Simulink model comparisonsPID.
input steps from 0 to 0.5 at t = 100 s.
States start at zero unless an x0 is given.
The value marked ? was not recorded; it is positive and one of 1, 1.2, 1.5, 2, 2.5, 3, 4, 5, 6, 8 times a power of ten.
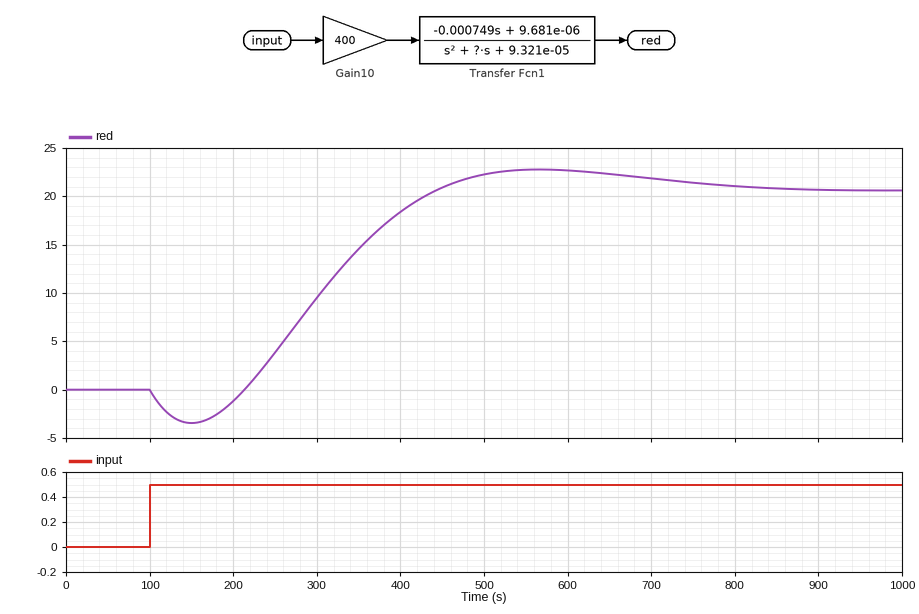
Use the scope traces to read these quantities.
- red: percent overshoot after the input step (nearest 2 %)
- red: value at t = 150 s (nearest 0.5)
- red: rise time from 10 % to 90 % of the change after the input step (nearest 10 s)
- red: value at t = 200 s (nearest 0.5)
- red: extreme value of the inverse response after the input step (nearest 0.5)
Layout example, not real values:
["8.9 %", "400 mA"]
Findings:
["10 %", "-3.5", "170 s", "-1.0", "-3.5"]
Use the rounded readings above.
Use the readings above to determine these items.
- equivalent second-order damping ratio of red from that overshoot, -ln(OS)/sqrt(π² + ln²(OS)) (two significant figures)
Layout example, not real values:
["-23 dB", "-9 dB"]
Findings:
["0.59"]
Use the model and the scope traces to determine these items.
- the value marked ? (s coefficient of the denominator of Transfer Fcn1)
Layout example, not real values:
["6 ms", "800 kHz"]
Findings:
["0.012"]
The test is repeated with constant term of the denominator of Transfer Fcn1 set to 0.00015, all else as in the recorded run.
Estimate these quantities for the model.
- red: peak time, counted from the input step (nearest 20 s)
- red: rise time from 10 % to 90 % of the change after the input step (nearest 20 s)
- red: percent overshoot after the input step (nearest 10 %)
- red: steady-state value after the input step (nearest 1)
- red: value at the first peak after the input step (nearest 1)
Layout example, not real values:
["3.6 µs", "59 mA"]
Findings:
["340 s", "100 s", "20 %", "13", "16"]
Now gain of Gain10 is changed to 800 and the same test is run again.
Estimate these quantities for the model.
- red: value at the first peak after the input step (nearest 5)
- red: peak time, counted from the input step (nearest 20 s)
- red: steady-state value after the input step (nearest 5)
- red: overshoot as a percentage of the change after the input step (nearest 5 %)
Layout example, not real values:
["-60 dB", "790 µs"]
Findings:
["45", "460 s", "40", "10 %"]
